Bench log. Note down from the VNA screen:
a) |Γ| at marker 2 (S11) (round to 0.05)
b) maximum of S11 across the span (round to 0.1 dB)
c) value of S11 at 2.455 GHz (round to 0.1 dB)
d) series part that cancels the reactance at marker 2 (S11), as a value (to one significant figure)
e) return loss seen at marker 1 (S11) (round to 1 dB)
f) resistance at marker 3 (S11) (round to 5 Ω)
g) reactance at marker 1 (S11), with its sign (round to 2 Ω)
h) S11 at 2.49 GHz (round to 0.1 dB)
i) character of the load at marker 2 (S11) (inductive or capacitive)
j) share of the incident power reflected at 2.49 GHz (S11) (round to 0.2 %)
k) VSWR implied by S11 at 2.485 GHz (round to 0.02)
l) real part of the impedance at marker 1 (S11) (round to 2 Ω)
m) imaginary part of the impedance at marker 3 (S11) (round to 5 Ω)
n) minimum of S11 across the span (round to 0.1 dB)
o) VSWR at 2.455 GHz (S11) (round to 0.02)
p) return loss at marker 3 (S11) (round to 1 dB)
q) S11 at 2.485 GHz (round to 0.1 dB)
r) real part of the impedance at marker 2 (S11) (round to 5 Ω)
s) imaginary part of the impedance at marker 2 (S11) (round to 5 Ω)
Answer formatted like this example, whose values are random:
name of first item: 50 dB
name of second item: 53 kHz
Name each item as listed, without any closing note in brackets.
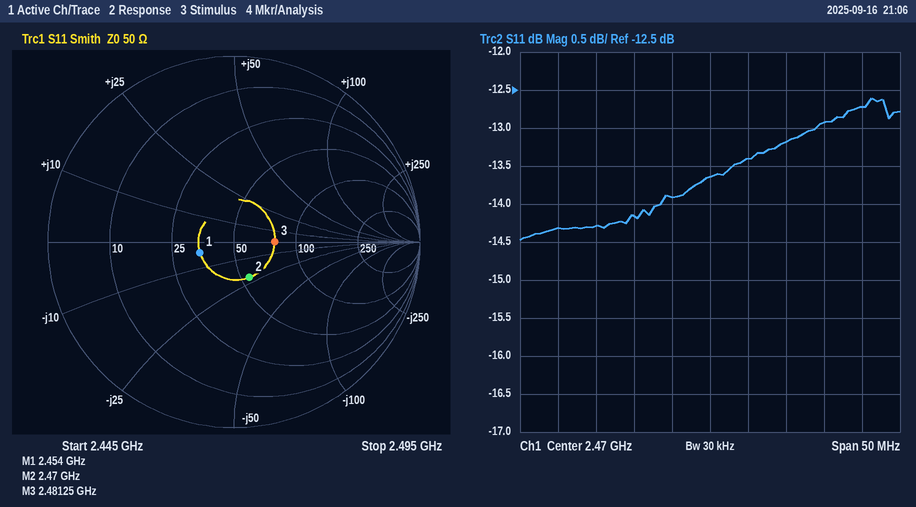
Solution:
|Γ| at marker 2 (S11): 0.20
maximum of S11 across the span: -12.6 dB
value of S11 at 2.455 GHz: -14.3 dB
series part that cancels the reactance at marker 2 (S11), as a value: 1 nH
return loss seen at marker 1 (S11): 14 dB
resistance at marker 3 (S11): 80 Ω
reactance at marker 1 (S11), with its sign: -4 Ω
S11 at 2.49 GHz: -12.7 dB
character of the load at marker 2 (S11): capacitive
share of the incident power reflected at 2.49 GHz (S11): 5.4 %
VSWR implied by S11 at 2.485 GHz: 1.58
real part of the impedance at marker 1 (S11): 34 Ω
imaginary part of the impedance at marker 3 (S11): 0 Ω
minimum of S11 across the span: -14.5 dB
VSWR at 2.455 GHz (S11): 1.48
return loss at marker 3 (S11): 13 dB
S11 at 2.485 GHz: -12.9 dB
real part of the impedance at marker 2 (S11): 55 Ω
imaginary part of the impedance at marker 2 (S11): -20 Ω
